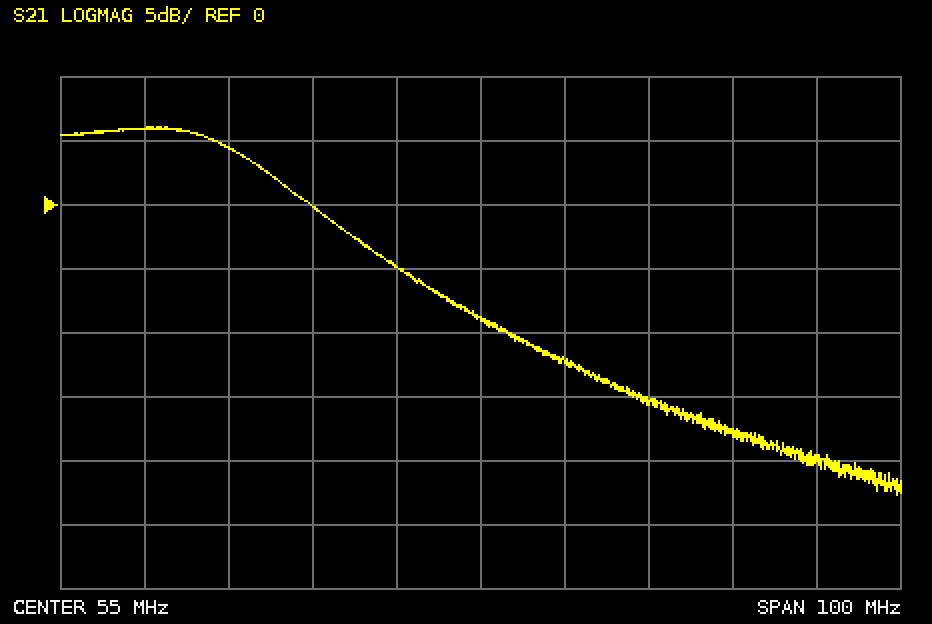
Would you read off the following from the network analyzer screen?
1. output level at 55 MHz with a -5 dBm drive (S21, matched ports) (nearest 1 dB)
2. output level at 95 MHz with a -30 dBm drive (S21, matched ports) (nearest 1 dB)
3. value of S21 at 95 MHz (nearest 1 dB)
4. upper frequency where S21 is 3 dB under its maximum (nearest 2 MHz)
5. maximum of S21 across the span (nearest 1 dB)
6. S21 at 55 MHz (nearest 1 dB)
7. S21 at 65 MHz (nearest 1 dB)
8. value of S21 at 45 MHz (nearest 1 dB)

-14 dBm
-50 dBm
-20 dB
28 MHz
6 dB
-9 dB
-12 dB
-5 dB
